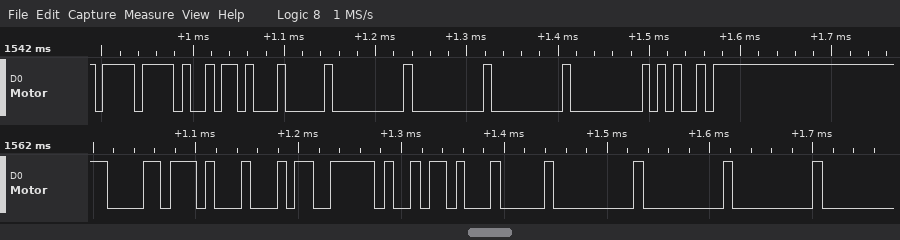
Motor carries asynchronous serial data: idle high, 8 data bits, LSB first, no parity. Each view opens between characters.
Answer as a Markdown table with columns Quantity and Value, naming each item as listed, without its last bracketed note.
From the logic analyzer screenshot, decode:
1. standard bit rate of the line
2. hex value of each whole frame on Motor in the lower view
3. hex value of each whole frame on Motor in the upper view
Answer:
| Quantity | Value |
|---|---|
| standard bit rate of the line | 115200 baud |
| hex value of each whole frame on Motor in the lower view | D8, 11, F3, 69, 04, 00, 00, 00 |
| hex value of each whole frame on Motor in the upper view | EF, 69, 04, 00, 00, 00, 00, A5 |
